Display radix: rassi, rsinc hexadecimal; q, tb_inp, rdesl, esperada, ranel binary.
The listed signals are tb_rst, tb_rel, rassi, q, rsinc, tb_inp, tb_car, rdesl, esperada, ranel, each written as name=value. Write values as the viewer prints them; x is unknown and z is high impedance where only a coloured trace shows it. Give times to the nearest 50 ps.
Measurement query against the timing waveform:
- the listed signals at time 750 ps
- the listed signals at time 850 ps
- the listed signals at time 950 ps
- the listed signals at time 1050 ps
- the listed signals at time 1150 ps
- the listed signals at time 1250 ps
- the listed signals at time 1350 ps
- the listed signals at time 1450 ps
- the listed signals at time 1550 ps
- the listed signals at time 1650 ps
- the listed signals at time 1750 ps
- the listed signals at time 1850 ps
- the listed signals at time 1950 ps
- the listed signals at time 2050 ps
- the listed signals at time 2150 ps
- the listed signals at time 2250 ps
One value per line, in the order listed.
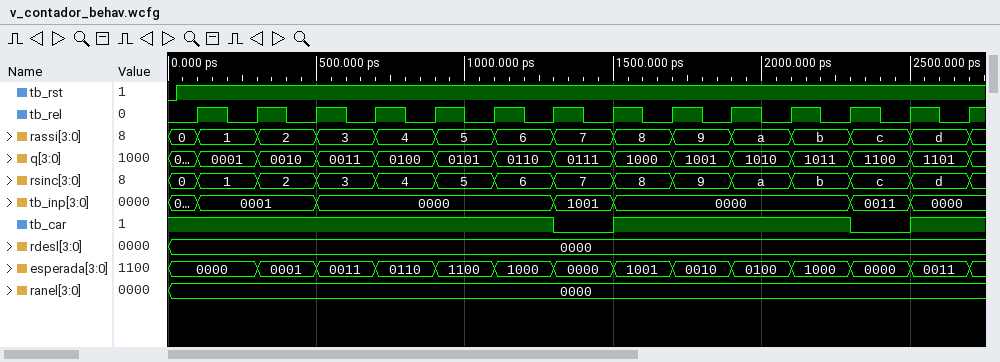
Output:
tb_rst=1, tb_rel=1, rassi=4, q=0100, rsinc=4, tb_inp=0000, tb_car=1, rdesl=0000, esperada=0110, ranel=0000
tb_rst=1, tb_rel=0, rassi=4, q=0100, rsinc=4, tb_inp=0000, tb_car=1, rdesl=0000, esperada=0110, ranel=0000
tb_rst=1, tb_rel=1, rassi=5, q=0101, rsinc=5, tb_inp=0000, tb_car=1, rdesl=0000, esperada=1100, ranel=0000
tb_rst=1, tb_rel=0, rassi=5, q=0101, rsinc=5, tb_inp=0000, tb_car=1, rdesl=0000, esperada=1100, ranel=0000
tb_rst=1, tb_rel=1, rassi=6, q=0110, rsinc=6, tb_inp=0000, tb_car=1, rdesl=0000, esperada=1000, ranel=0000
tb_rst=1, tb_rel=0, rassi=6, q=0110, rsinc=6, tb_inp=0000, tb_car=1, rdesl=0000, esperada=1000, ranel=0000
tb_rst=1, tb_rel=1, rassi=7, q=0111, rsinc=7, tb_inp=1001, tb_car=0, rdesl=0000, esperada=0000, ranel=0000
tb_rst=1, tb_rel=0, rassi=7, q=0111, rsinc=7, tb_inp=1001, tb_car=0, rdesl=0000, esperada=0000, ranel=0000
tb_rst=1, tb_rel=1, rassi=8, q=1000, rsinc=8, tb_inp=0000, tb_car=1, rdesl=0000, esperada=1001, ranel=0000
tb_rst=1, tb_rel=0, rassi=8, q=1000, rsinc=8, tb_inp=0000, tb_car=1, rdesl=0000, esperada=1001, ranel=0000
tb_rst=1, tb_rel=1, rassi=9, q=1001, rsinc=9, tb_inp=0000, tb_car=1, rdesl=0000, esperada=0010, ranel=0000
tb_rst=1, tb_rel=0, rassi=9, q=1001, rsinc=9, tb_inp=0000, tb_car=1, rdesl=0000, esperada=0010, ranel=0000
tb_rst=1, tb_rel=1, rassi=a, q=1010, rsinc=a, tb_inp=0000, tb_car=1, rdesl=0000, esperada=0100, ranel=0000
tb_rst=1, tb_rel=0, rassi=a, q=1010, rsinc=a, tb_inp=0000, tb_car=1, rdesl=0000, esperada=0100, ranel=0000
tb_rst=1, tb_rel=1, rassi=b, q=1011, rsinc=b, tb_inp=0000, tb_car=1, rdesl=0000, esperada=1000, ranel=0000
tb_rst=1, tb_rel=0, rassi=b, q=1011, rsinc=b, tb_inp=0000, tb_car=1, rdesl=0000, esperada=1000, ranel=0000
